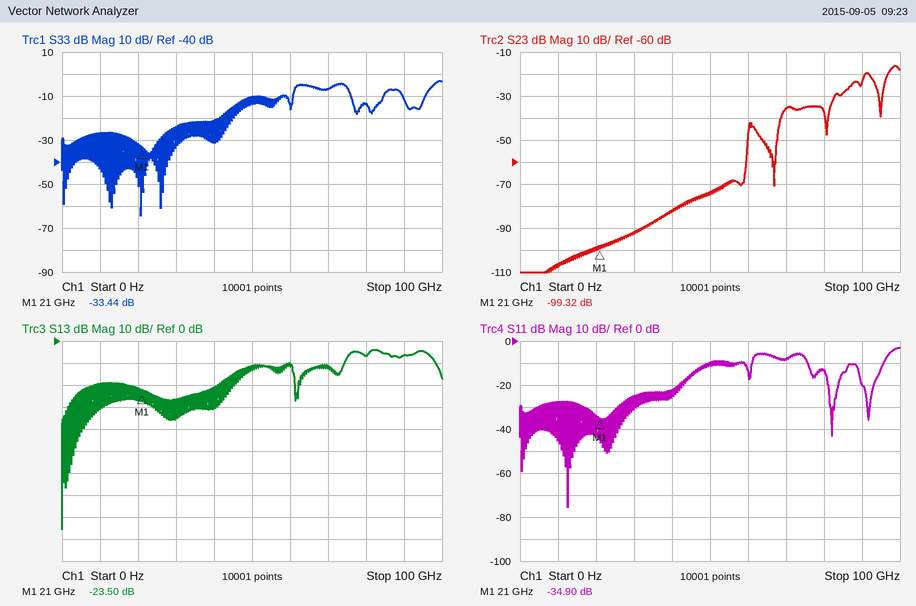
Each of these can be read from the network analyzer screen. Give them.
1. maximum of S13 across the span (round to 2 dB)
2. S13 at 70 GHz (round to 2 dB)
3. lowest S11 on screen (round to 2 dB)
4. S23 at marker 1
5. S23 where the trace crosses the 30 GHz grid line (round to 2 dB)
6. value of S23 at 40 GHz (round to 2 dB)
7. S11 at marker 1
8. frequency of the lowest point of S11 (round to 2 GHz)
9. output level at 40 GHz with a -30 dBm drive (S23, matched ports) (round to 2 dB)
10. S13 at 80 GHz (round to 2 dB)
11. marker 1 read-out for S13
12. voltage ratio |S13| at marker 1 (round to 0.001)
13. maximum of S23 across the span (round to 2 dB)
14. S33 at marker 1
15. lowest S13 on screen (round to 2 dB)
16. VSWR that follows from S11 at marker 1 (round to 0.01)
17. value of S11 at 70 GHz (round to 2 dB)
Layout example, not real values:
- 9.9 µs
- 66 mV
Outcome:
- -4 dB
- -12 dB
- -76 dB
- -99.32 dB
- -92 dB
- -82 dB
- -34.90 dB
- 12 GHz
- -112 dBm
- -6 dB
- -23.50 dB
- 0.067
- -16 dB
- -33.44 dB
- -86 dB
- 1.04
- -8 dB
